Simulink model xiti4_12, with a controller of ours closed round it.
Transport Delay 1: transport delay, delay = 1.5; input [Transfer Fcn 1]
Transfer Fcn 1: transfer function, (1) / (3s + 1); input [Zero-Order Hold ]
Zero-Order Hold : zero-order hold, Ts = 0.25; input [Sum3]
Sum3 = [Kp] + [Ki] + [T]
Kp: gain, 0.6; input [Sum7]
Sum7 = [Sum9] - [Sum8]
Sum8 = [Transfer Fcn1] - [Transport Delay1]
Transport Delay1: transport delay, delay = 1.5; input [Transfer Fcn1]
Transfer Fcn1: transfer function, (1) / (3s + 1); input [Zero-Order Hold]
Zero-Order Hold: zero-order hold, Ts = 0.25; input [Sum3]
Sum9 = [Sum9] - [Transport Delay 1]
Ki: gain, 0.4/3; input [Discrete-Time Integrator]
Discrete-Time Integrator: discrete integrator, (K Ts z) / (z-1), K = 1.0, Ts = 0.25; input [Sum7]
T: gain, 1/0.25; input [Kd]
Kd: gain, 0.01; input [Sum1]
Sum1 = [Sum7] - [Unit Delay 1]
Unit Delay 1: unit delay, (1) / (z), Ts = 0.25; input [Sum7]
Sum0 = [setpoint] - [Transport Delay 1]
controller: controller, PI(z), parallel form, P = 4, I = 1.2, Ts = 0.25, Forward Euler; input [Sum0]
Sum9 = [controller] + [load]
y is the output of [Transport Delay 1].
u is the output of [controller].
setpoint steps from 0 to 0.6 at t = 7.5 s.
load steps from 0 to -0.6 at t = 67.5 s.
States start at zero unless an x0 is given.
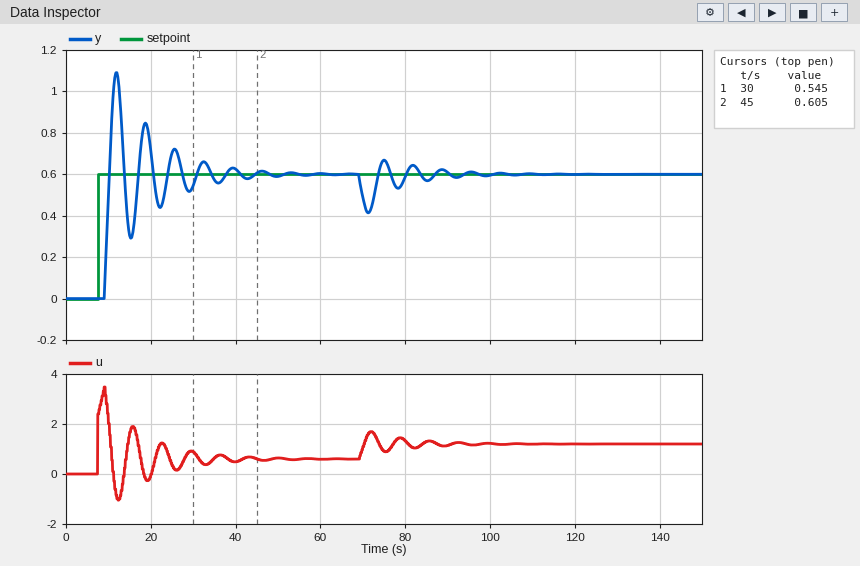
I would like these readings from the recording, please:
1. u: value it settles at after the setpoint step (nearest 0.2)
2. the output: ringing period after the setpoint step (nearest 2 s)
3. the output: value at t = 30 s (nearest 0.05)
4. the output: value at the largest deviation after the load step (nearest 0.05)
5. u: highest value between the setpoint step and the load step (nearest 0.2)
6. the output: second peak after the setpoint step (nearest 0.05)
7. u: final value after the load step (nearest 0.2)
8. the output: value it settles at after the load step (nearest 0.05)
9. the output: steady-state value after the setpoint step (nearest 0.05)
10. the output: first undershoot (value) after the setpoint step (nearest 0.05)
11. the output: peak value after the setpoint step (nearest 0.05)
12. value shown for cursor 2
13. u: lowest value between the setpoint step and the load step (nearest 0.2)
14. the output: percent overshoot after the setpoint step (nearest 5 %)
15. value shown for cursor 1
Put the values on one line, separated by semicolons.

0.6; 6 s; 0.55; 0.40; 3.4; 0.85; 1.2; 0.60; 0.60; 0.30; 1.10; 0.605; -1.0; 80 %; 0.545
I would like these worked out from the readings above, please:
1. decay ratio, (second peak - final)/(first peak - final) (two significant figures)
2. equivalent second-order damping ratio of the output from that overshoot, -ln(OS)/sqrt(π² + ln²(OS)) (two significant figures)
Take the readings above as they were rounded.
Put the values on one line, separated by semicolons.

0.50; 0.071
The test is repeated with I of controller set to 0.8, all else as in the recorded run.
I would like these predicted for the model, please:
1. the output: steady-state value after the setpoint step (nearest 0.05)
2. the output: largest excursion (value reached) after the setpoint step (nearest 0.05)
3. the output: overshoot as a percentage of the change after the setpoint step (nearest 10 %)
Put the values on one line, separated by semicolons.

0.60; 0.95; 60 %
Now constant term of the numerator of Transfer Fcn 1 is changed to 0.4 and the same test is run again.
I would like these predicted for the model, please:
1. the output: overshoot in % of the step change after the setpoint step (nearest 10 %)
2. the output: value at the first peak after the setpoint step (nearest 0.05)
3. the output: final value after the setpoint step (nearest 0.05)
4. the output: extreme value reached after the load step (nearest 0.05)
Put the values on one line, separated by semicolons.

40 %; 0.80; 0.60; 0.50
